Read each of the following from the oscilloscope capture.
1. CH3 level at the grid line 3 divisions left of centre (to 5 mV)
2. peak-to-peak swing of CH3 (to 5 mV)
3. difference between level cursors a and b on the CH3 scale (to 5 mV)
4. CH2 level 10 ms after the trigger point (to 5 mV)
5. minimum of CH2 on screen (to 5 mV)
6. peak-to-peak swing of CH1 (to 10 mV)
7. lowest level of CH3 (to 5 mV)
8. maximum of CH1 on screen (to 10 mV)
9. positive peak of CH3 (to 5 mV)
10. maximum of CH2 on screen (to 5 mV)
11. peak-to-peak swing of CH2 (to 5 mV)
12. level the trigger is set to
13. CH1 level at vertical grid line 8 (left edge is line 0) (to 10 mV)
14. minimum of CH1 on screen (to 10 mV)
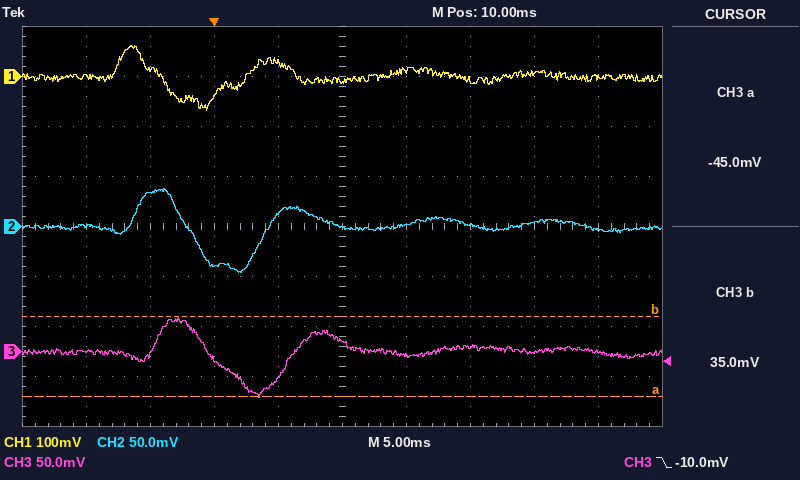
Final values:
0 mV
80 mV
80 mV
0 mV
-45 mV
130 mV
-45 mV
60 mV
35 mV
40 mV
85 mV
-10.0 mV
10 mV
-70 mV
